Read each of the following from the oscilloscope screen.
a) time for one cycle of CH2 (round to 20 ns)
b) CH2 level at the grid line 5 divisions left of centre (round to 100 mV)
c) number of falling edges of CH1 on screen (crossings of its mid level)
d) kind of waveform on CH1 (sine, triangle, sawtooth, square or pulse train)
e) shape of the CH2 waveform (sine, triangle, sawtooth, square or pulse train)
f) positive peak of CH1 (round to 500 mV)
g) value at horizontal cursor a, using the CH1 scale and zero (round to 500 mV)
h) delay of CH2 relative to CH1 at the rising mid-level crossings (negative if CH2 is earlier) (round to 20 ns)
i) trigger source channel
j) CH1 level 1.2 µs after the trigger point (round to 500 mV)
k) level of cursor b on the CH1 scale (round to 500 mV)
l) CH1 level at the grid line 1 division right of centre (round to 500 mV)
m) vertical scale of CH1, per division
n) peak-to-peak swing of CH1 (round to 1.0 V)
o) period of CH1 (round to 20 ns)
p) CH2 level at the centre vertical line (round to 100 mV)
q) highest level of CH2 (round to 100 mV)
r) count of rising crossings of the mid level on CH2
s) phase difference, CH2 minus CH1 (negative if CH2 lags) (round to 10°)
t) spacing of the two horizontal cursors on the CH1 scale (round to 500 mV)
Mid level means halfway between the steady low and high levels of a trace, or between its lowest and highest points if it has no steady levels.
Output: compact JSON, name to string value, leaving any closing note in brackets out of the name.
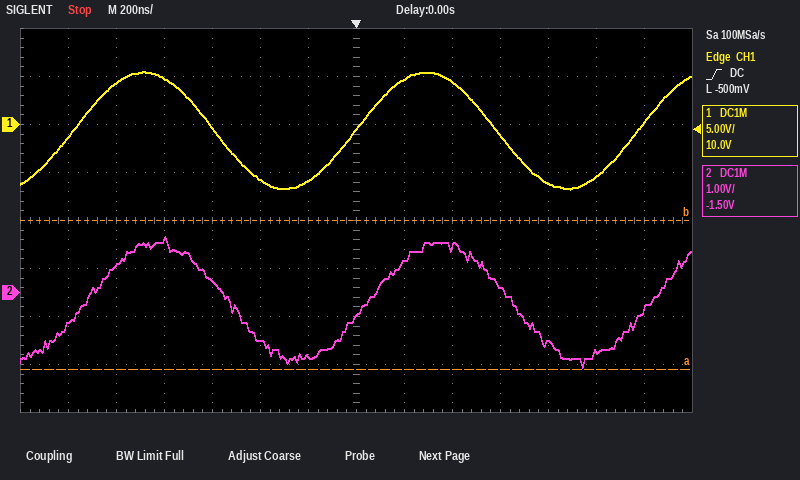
{"time for one cycle of CH2": "1.18 µs", "CH2 level at the grid line 5 divisions left of centre": "600 mV", "number of falling edges of CH1 on screen": "2", "kind of waveform on CH1": "sine", "shape of the CH2 waveform": "sine", "positive peak of CH1": "5.5 V", "value at horizontal cursor a, using the CH1 scale and zero": "-25.5 V", "delay of CH2 relative to CH1 at the rising mid-level crossings (negative if CH2 is earlier)": "+60 ns", "trigger source channel": "CH1", "CH1 level 1.2 µs after the trigger point": "0.0 V", "level of cursor b on the CH1 scale": "-10.0 V", "CH1 level at the grid line 1 division right of centre": "4.5 V", "vertical scale of CH1, per division": "5 V", "peak-to-peak swing of CH1": "12.0 V", "period of CH1": "1.18 µs", "CH2 level at the centre vertical line": "-500 mV", "highest level of CH2": "1.2 V", "count of rising crossings of the mid level on CH2": "3", "phase difference, CH2 minus CH1 (negative if CH2 lags)": "-20°", "spacing of the two horizontal cursors on the CH1 scale": "15.5 V"}
